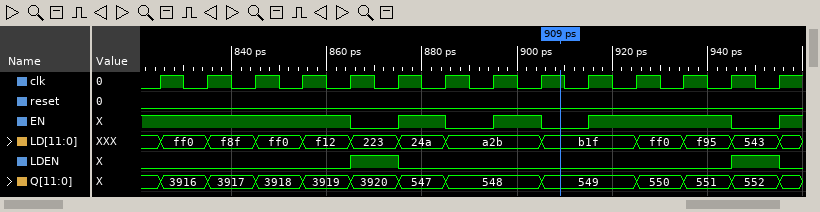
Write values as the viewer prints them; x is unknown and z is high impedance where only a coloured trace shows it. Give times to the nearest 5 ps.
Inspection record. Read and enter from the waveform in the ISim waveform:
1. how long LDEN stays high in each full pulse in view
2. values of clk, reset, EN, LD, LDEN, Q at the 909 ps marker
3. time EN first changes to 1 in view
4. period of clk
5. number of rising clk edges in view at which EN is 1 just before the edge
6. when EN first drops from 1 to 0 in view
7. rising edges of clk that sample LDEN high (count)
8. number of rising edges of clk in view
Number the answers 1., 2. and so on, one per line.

1. 10 ps, 10 ps
2. clk=1, reset=0, EN=0, LD=b1f, LDEN=0, Q=549
3. 875 ps
4. 10 ps
5. 10
6. 865 ps
7. 2
8. 14
